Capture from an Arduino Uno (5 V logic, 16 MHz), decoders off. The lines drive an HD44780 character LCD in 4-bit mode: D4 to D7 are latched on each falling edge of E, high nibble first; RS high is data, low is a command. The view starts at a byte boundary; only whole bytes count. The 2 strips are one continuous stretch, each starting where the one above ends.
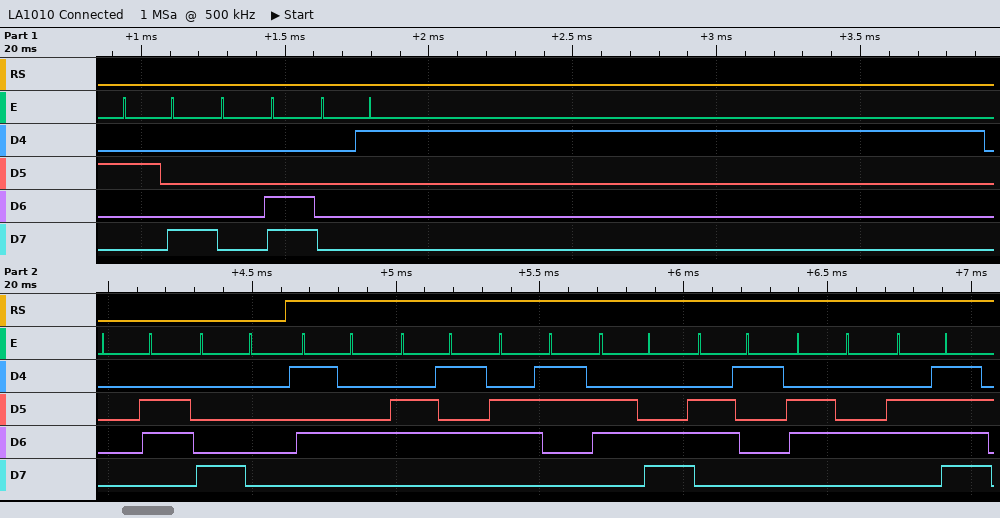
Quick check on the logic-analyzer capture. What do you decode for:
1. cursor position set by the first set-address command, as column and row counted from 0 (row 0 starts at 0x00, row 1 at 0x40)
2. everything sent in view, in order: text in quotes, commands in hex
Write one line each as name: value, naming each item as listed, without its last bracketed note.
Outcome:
cursor position set by the first set-address command, as column and row counted from 0: column 0, row 0
everything sent in view, in order: text in quotes, commands in hex: 0x28 0x0C 0x01 0x06 0x80 "Teclado"
